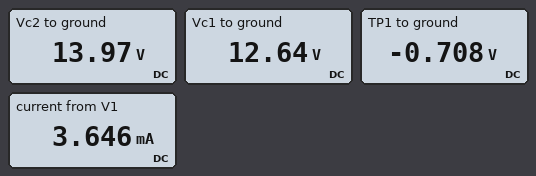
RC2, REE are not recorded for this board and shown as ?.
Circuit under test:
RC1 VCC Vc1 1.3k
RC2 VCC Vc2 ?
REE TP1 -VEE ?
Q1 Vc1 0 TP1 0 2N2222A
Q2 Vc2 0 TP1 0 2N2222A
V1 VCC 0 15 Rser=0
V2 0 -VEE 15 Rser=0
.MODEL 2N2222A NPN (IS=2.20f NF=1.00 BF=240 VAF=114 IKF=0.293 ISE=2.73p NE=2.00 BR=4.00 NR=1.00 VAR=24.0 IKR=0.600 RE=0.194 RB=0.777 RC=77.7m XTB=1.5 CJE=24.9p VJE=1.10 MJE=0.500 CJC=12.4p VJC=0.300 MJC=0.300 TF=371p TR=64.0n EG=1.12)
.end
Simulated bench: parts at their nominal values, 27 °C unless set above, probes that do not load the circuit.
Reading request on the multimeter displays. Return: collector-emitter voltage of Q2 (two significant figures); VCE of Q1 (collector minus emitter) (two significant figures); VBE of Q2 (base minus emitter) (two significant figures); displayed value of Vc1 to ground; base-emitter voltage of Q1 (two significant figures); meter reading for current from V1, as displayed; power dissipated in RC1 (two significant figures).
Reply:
15 V
13 V
710 mV
12.64 V
710 mV
3.646 mA
4.3 mW
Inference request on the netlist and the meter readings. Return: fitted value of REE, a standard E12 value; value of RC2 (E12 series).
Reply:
3.9 kΩ
560 Ω
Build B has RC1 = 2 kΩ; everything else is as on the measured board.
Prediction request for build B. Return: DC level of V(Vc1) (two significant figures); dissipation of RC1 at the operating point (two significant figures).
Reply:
11 V
6.5 mW
